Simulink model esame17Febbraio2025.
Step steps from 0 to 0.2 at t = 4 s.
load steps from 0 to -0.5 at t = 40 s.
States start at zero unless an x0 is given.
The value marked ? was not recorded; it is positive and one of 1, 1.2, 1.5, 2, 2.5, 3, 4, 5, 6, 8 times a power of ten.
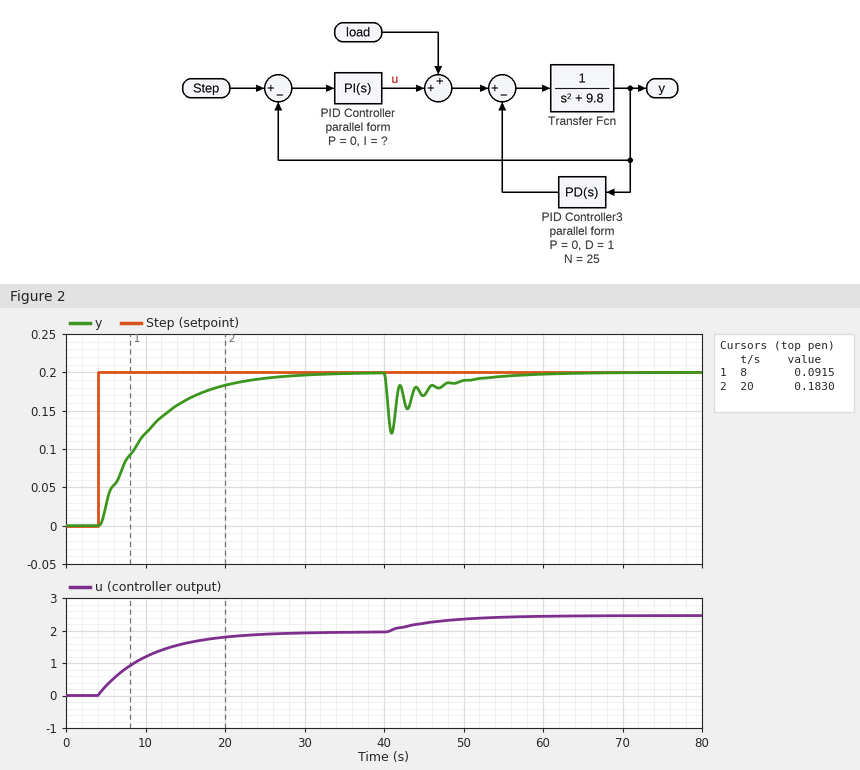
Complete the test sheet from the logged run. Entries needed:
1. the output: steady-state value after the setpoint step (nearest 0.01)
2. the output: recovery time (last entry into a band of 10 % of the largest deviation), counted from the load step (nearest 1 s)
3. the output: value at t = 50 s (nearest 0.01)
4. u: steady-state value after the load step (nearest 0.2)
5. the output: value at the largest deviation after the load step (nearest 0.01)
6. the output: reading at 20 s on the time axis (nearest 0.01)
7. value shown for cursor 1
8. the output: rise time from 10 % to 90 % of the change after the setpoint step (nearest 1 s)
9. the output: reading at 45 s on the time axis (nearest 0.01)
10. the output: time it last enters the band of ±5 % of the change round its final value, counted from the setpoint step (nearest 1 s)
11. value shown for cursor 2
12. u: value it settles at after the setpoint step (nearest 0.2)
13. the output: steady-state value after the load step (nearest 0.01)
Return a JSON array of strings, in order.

["0.20", "12 s", "0.19", "2.4", "0.12", "0.18", "0.0915", "14 s", "0.17", "19 s", "0.1830", "2.0", "0.20"]
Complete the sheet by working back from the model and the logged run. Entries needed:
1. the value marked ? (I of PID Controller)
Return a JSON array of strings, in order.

["1.5"]
